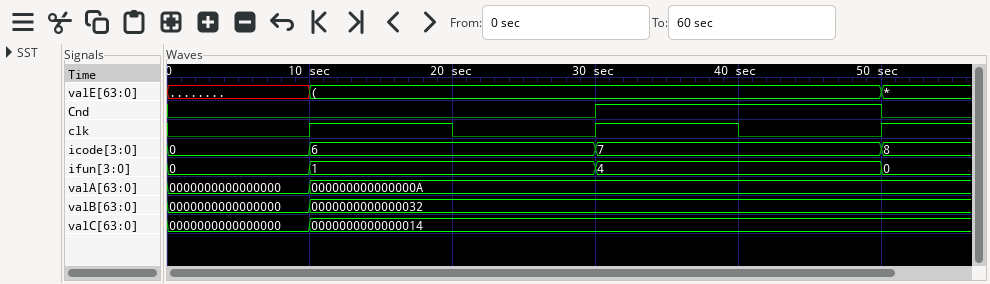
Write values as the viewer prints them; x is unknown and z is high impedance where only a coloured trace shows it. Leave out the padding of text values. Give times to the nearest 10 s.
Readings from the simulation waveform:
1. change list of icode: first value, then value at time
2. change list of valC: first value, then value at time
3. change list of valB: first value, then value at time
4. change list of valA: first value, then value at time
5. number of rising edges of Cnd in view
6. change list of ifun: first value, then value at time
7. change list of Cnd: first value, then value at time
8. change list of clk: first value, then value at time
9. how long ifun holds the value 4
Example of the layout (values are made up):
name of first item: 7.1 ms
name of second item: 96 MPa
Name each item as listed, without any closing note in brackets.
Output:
change list of icode: first value, then value at time: 0, 6 at 10 s, 7 at 30 s, 8 at 50 s
change list of valC: first value, then value at time: 0000000000000000, 0000000000000014 at 10 s
change list of valB: first value, then value at time: 0000000000000000, 0000000000000032 at 10 s
change list of valA: first value, then value at time: 0000000000000000, 000000000000000A at 10 s
number of rising edges of Cnd in view: 1
change list of ifun: first value, then value at time: 0, 1 at 10 s, 4 at 30 s, 0 at 50 s
change list of Cnd: first value, then value at time: 0, 1 at 30 s, 0 at 50 s
change list of clk: first value, then value at time: 0, 1 at 10 s, 0 at 20 s, 1 at 30 s, 0 at 40 s, 1 at 50 s
how long ifun holds the value 4: 20 s
